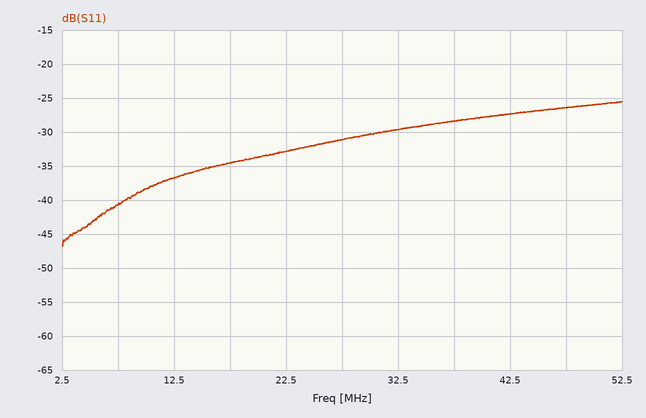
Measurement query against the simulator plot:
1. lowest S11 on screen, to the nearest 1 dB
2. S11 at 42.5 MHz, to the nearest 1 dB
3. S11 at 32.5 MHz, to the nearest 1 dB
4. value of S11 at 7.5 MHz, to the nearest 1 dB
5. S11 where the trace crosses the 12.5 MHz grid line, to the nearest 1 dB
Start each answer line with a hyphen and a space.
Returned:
- -47 dB
- -27 dB
- -30 dB
- -41 dB
- -37 dB
